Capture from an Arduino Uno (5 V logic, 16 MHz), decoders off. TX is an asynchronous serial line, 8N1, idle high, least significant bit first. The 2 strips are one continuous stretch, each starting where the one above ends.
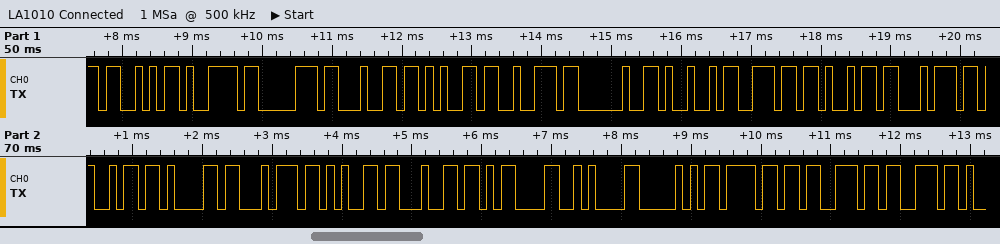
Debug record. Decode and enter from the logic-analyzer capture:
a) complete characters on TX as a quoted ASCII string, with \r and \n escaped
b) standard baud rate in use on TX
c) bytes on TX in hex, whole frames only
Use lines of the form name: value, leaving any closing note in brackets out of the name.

complete characters on TX as a quoted ASCII string, with \r and \n escaped: "Sypder Initiated\r\nPoss"
standard baud rate in use on TX: 9600 baud
bytes on TX in hex, whole frames only: 0x53 0x79 0x70 0x64 0x65 0x72 0x20 0x49 0x6E 0x69 0x74 0x69 0x61 0x74 0x65 0x64 0x0D 0x0A 0x50 0x6F 0x73 0x73
